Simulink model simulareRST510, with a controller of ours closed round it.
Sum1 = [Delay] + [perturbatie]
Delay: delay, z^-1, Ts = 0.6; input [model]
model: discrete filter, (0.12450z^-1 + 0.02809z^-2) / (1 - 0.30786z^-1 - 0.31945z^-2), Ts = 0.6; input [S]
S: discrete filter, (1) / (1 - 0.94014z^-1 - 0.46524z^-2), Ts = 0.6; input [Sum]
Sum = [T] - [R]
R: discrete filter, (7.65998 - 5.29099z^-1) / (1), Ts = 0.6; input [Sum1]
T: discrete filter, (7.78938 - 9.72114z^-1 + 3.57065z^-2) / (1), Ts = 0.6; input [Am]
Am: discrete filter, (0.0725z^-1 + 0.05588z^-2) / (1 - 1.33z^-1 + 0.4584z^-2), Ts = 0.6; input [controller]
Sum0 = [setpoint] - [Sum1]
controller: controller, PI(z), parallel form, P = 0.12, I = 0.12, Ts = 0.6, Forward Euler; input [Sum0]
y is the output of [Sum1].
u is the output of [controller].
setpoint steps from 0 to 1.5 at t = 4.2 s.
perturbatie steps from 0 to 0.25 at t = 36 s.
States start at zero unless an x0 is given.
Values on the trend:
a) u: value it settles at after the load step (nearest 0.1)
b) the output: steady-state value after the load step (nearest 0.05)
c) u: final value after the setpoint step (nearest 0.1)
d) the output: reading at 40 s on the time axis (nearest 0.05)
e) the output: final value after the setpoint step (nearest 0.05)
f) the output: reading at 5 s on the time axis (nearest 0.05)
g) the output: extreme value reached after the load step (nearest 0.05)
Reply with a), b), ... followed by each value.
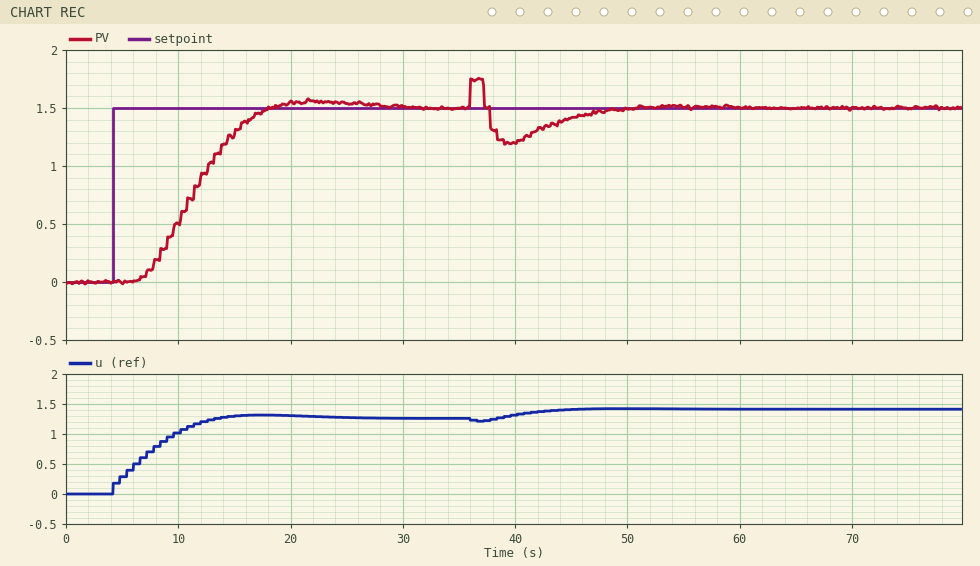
a) 1.4
b) 1.50
c) 1.3
d) 1.20
e) 1.50
f) 0.00
g) 1.20
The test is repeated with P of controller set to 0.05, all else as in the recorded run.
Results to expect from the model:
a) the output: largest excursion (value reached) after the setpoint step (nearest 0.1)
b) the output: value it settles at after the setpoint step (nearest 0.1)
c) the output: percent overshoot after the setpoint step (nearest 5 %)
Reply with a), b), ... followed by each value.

a) 1.6
b) 1.5
c) 10 %
